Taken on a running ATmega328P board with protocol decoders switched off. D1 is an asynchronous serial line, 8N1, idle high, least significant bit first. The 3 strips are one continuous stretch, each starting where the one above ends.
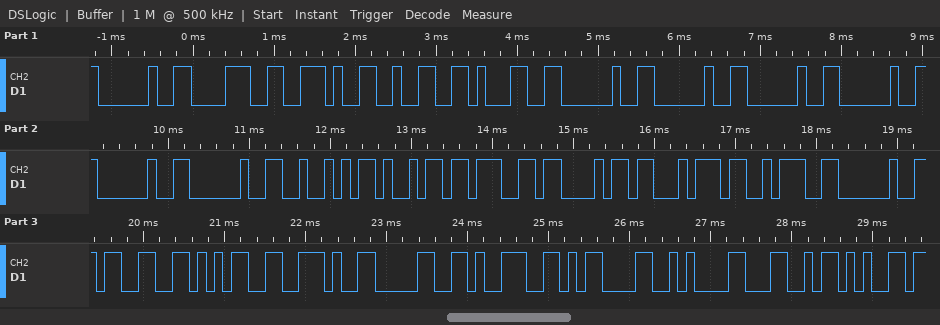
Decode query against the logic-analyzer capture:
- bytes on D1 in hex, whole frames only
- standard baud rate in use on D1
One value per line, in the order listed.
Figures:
20 38 2E 32 31 20 20 20 20 20 20 52 69 67 68 74 3A 20 33 35 2E 30 39 0D 0A 4C 65
9600 baud
